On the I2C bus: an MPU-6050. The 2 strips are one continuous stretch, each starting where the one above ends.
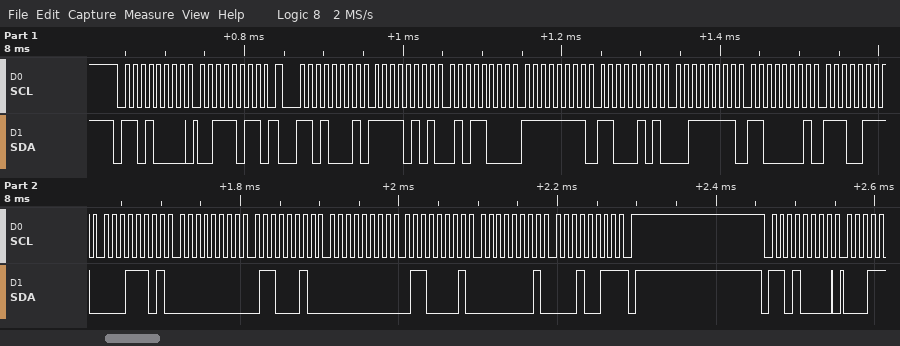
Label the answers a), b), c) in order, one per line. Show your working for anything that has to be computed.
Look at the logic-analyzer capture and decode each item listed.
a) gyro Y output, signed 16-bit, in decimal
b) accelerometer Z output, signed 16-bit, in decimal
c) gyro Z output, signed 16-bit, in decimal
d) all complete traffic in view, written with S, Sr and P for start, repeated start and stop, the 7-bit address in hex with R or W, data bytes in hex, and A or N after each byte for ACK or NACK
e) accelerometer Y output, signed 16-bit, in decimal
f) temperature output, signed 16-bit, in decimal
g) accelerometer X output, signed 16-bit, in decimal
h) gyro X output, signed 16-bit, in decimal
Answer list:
a) 0x0061 = 97
b) 0x3FC1 = 16321
c) 0x0113 = 275
d) S 68W A 3B A Sr 68R A F5 A 58 A FF A C5 A 3F A C1 A E7 A 1D A 00 A 62 A 00 A 61 A 01 A 13 N P S 68W A
e) 0xFFC5 = -59
f) 0xE71D = -6371
g) 0xF558 = -2728
h) 0x0062 = 98
